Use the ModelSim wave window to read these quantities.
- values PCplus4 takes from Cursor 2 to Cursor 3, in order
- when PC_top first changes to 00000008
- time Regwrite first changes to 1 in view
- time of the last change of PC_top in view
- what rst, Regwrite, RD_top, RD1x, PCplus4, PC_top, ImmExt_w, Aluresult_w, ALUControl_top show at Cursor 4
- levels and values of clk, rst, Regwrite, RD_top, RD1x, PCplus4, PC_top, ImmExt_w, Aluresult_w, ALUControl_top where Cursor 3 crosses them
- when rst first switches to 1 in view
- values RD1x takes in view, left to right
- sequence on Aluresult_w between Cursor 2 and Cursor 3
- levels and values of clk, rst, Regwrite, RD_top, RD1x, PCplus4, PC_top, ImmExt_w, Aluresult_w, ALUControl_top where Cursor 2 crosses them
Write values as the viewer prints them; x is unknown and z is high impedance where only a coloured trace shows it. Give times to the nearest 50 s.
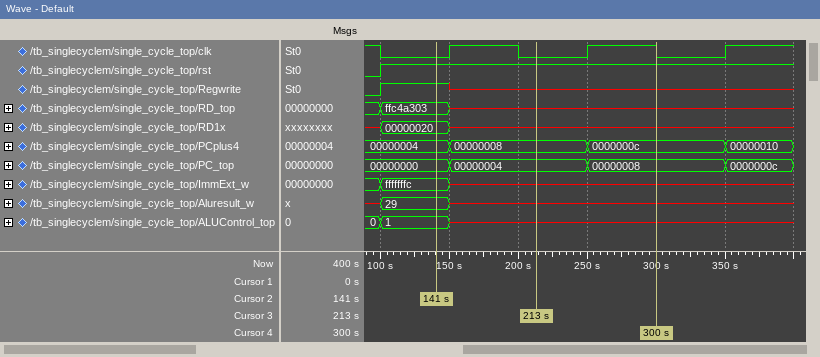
00000004, 00000008
250 s
100 s
350 s
rst=1, Regwrite=x, RD_top=x, RD1x=x, PCplus4=0000000c, PC_top=00000008, ImmExt_w=x, Aluresult_w=x, ALUControl_top=x
clk=0, rst=1, Regwrite=x, RD_top=x, RD1x=x, PCplus4=00000008, PC_top=00000004, ImmExt_w=x, Aluresult_w=x, ALUControl_top=x
100 s
x, 00000020, x
29, x
clk=0, rst=1, Regwrite=1, RD_top=ffc4a303, RD1x=00000020, PCplus4=00000004, PC_top=00000000, ImmExt_w=fffffffc, Aluresult_w=29, ALUControl_top=1
